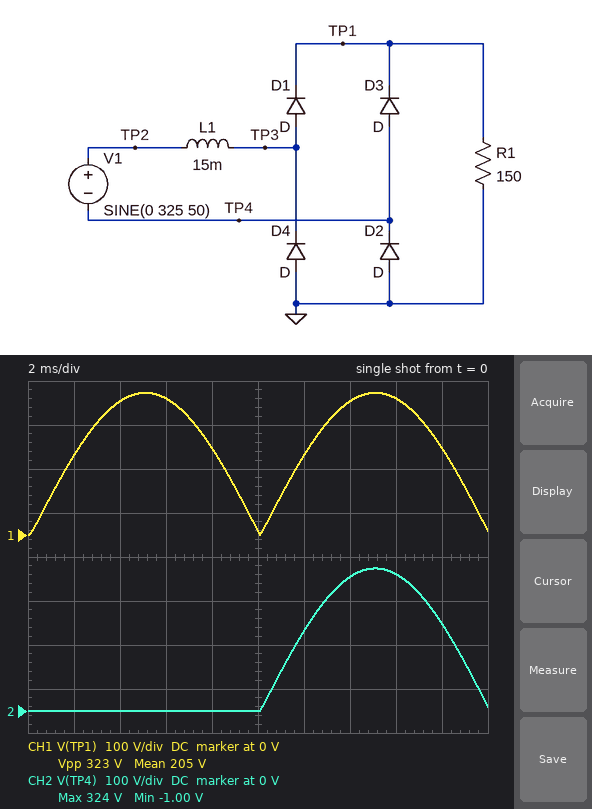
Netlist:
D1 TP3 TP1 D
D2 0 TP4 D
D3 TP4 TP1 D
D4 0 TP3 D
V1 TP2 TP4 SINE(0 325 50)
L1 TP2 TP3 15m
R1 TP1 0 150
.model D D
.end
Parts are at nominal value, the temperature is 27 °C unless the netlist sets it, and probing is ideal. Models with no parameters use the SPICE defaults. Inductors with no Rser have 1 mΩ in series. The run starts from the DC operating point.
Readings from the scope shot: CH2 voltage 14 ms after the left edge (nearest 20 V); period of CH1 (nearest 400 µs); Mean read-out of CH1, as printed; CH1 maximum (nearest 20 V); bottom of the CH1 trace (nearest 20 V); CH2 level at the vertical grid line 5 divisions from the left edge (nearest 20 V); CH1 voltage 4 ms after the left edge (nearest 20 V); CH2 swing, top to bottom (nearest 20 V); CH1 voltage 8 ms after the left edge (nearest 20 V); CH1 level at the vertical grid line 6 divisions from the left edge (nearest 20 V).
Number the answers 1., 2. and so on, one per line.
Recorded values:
1. 300 V
2. 10.0 ms
3. 205 V
4. 320 V
5. 0 V
6. 0 V
7. 300 V
8. 320 V
9. 200 V
10. 180 V
